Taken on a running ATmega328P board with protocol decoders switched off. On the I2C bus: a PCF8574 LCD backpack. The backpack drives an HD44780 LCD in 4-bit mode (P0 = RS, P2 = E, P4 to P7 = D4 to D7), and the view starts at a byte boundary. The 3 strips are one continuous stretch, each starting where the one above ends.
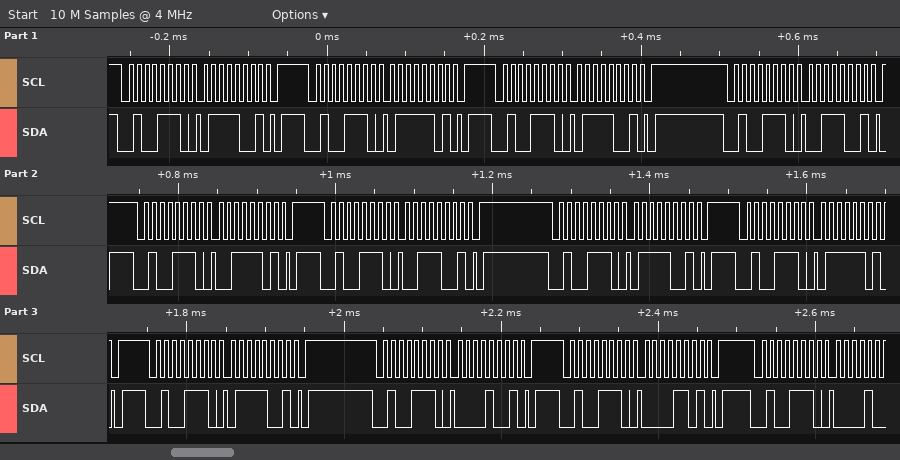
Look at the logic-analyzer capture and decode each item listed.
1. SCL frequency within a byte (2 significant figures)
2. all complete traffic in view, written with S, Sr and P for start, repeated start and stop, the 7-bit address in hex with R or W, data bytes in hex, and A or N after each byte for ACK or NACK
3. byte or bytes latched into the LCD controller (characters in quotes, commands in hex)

100 kHz
S 27W A 79 A P S 27W A 7D A P S 27W A 79 A P S 27W A 39 A P S 27W A 3D A P S 27W A 39 A P S 27W A 79 A P S 27W A 7D A P S 27W A 79 A P S 27W A 09 A P S 27W A 0D A P S 27W A
's'
